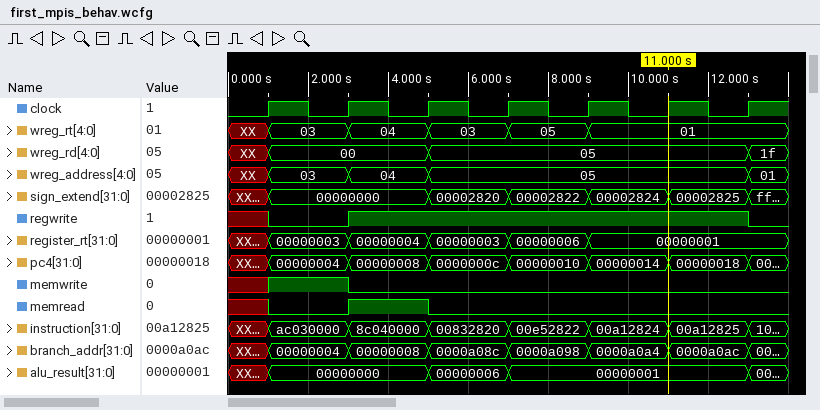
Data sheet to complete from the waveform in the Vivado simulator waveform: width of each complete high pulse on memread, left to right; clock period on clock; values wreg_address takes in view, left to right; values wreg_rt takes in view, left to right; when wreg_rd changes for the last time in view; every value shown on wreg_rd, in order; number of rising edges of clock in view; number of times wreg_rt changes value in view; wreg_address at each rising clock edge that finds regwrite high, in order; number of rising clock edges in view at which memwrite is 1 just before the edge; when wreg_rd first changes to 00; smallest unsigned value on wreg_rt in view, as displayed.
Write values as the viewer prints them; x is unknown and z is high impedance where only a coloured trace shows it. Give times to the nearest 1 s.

2 s
2 s
XX, 03, 04, 05, 01
XX, 03, 04, 03, 05, 01
13 s
XX, 00, 05, 1f
7
5
04, 05, 05, 05, 05
1
1 s
01
